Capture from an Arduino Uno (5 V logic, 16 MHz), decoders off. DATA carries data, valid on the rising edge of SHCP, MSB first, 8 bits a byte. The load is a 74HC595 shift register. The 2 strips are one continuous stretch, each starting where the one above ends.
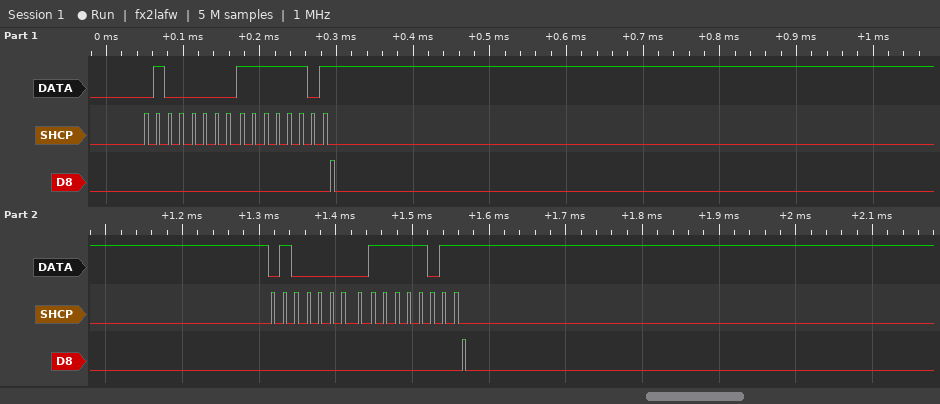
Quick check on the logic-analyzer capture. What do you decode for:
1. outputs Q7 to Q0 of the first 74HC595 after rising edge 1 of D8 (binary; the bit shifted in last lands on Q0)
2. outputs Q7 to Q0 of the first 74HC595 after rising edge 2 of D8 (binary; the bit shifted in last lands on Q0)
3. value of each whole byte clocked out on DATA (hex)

11111101
11111011
40 FD 40 FB
